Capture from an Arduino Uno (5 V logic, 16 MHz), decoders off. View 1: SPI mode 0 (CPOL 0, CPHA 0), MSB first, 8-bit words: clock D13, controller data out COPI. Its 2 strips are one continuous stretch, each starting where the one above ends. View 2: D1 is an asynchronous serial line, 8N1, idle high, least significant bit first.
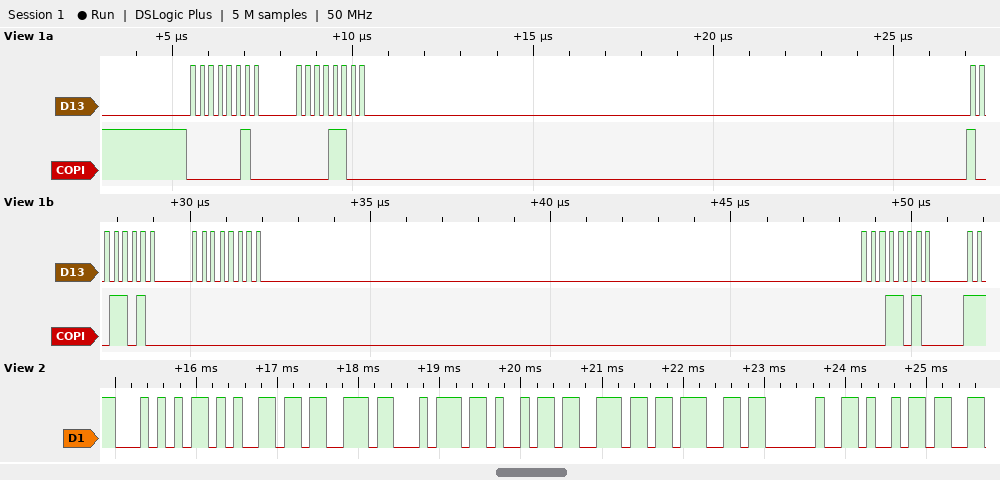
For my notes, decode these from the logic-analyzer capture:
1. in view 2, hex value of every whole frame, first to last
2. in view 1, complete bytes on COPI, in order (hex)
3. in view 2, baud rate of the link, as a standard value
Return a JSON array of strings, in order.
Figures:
["54 65 73 74 69 6E 67 20 69", "0x02 0x0C 0x9A 0x00 0x1A", "9600 baud"]
